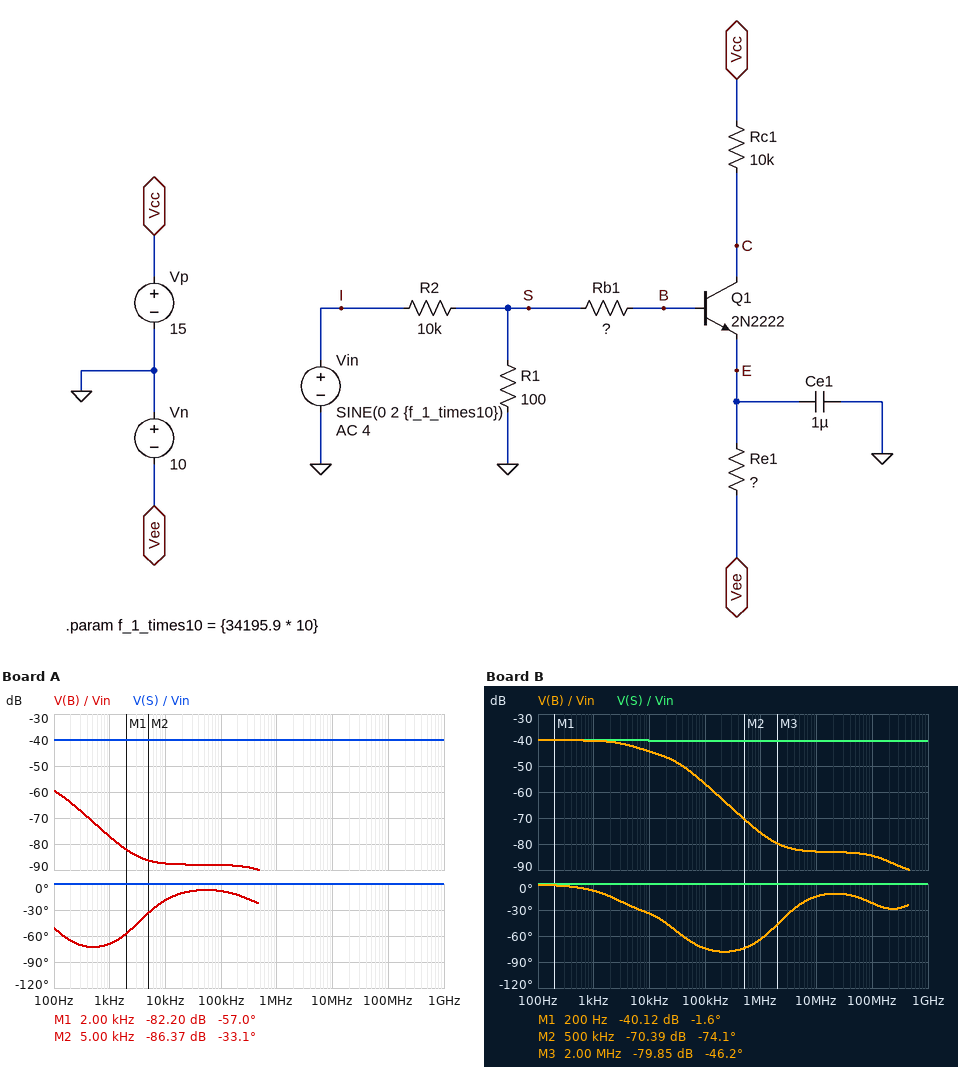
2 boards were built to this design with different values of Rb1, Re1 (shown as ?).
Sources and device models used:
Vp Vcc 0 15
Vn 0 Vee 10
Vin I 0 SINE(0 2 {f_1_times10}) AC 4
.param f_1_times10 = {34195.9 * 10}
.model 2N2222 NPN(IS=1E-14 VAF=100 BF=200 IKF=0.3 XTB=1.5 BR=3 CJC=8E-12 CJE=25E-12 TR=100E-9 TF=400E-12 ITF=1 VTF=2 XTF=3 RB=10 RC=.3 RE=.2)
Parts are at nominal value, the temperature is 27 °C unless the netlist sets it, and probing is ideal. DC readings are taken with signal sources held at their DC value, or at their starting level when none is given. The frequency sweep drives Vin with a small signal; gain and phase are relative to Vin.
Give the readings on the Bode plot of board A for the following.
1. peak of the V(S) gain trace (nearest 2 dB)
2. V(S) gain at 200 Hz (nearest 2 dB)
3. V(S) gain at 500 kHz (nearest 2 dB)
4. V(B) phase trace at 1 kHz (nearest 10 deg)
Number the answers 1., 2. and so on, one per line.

1. -40 dB
2. -40 dB
3. -40 dB
4. -70 deg
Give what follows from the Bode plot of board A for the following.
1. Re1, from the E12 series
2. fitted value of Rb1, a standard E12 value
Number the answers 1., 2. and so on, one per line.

1. 3.3 kΩ
2. 12 kΩ
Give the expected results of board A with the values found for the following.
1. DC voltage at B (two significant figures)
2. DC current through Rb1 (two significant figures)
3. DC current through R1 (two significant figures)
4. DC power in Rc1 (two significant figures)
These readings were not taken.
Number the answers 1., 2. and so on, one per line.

1. -2.6 V
2. 210 µA
3. 210 µA
4. 33 mW
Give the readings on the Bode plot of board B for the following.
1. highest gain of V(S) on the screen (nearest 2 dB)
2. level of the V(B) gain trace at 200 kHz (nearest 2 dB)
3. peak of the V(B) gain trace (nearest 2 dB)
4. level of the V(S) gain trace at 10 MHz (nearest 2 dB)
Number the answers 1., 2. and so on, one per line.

1. -40 dB
2. -62 dB
3. -40 dB
4. -40 dB
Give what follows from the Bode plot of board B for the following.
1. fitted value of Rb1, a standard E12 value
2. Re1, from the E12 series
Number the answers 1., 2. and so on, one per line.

1. 3.9 kΩ
2. 6.8 kΩ
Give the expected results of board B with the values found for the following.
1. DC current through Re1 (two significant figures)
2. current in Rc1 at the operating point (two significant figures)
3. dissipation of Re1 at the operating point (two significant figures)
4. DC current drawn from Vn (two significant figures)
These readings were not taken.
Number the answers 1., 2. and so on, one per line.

1. 1.4 mA
2. 1.4 mA
3. 13 mW
4. 1.4 mA
